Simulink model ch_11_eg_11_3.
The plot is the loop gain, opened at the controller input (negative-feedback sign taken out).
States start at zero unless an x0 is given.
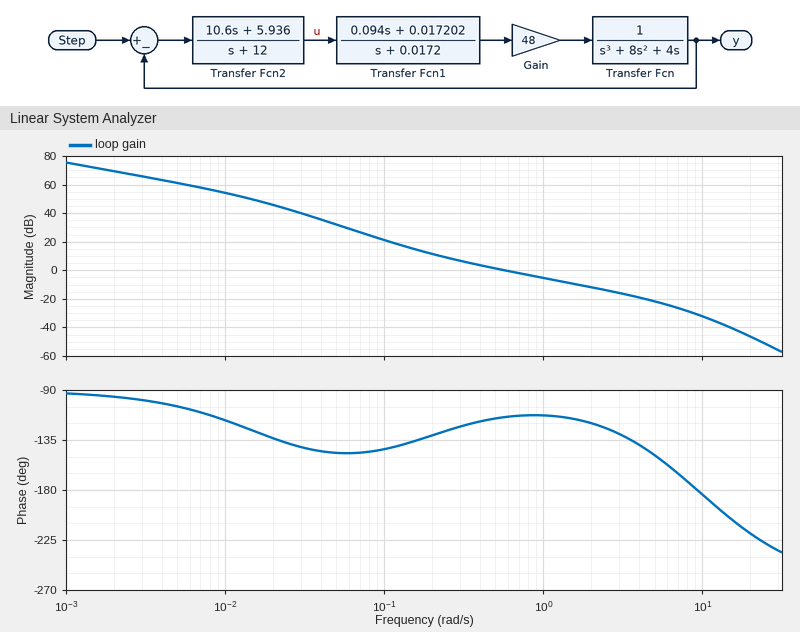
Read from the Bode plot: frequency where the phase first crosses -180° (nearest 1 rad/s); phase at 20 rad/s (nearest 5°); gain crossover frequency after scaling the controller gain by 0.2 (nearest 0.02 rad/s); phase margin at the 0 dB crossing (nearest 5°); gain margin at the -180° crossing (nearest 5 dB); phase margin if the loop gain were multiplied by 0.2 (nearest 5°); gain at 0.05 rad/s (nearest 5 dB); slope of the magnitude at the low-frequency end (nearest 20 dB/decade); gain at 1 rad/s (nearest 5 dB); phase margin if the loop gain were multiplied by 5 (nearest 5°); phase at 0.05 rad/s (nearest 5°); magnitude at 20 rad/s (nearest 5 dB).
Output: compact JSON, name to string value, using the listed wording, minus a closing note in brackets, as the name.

{"frequency where the phase first crosses -180°": "9 rad/s", "phase at 20 rad/s": "-220°", "gain crossover frequency after scaling the controller gain by 0.2": "0.16 rad/s", "phase margin at the 0 dB crossing": "65°", "gain margin at the -180° crossing": "30 dB", "phase margin if the loop gain were multiplied by 0.2": "45°", "gain at 0.05 rad/s": "30 dB", "slope of the magnitude at the low-frequency end": "-20 dB/decade", "gain at 1 rad/s": "-5 dB", "phase margin if the loop gain were multiplied by 5": "55°", "phase at 0.05 rad/s": "-145°", "magnitude at 20 rad/s": "-45 dB"}
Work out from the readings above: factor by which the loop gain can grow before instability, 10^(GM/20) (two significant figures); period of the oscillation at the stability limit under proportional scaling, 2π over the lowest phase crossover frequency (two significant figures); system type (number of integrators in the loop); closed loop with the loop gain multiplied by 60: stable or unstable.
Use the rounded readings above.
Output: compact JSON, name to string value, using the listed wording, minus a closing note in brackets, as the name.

{"factor by which the loop gain can grow before instability, 10^(GM/20)": "32", "period of the oscillation at the stability limit under proportional scaling, 2π over the lowest phase crossover frequency": "0.70 s", "system type": "1", "closed loop with the loop gain multiplied by 60: stable or unstable": "unstable"}
